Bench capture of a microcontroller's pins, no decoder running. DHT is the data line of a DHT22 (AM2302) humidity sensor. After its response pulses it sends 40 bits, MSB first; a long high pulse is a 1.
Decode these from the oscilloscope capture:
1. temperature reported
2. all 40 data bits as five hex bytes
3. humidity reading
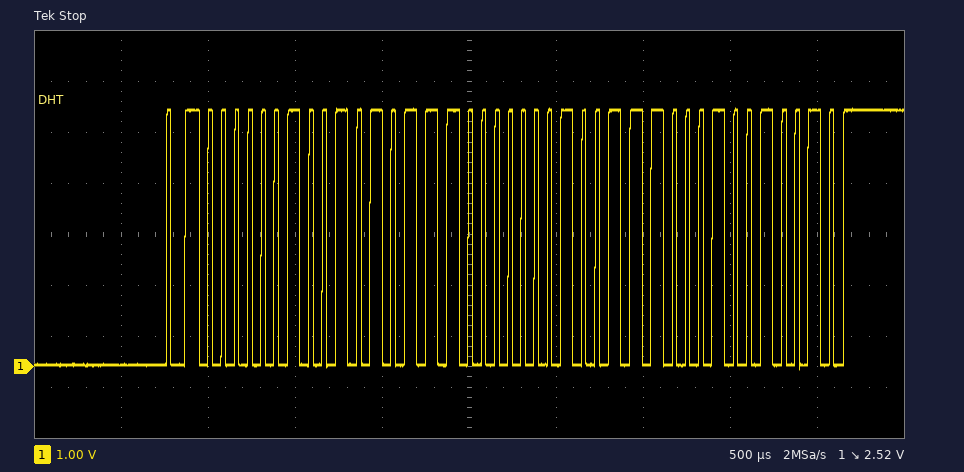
31.2 °C
02 57 01 38 92
59.9 %
